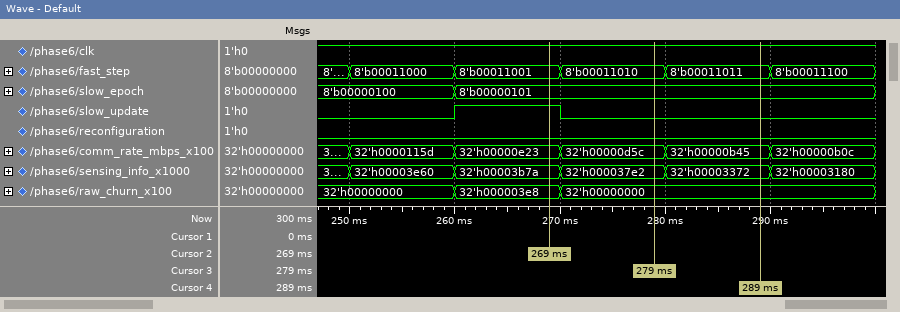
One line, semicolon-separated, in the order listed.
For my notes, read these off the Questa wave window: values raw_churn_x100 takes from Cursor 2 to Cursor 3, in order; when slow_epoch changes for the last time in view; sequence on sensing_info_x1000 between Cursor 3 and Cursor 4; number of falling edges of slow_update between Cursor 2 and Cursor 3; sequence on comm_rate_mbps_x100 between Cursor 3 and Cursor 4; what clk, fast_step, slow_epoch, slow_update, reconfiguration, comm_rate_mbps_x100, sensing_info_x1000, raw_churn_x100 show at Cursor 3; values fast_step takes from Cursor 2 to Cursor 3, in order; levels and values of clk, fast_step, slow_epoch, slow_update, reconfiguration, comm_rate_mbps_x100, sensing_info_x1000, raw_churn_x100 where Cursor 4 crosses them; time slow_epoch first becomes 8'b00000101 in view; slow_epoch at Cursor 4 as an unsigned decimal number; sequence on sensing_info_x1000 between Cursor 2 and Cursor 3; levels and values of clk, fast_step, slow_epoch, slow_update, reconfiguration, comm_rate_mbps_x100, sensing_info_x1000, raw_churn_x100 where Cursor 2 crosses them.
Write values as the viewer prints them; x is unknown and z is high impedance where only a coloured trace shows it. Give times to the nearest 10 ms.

32'h000003e8, 32'h00000000; 260 ms; 32'h000037e2, 32'h00003372; 1; 32'h00000d5c, 32'h00000b45; clk=1, fast_step=8'b00011010, slow_epoch=8'b00000101, slow_update=0, reconfiguration=0, comm_rate_mbps_x100=32'h00000d5c, sensing_info_x1000=32'h000037e2, raw_churn_x100=32'h00000000; 8'b00011001, 8'b00011010; clk=1, fast_step=8'b00011011, slow_epoch=8'b00000101, slow_update=0, reconfiguration=0, comm_rate_mbps_x100=32'h00000b45, sensing_info_x1000=32'h00003372, raw_churn_x100=32'h00000000; 260 ms; 5; 32'h00003b7a, 32'h000037e2; clk=1, fast_step=8'b00011001, slow_epoch=8'b00000101, slow_update=1, reconfiguration=0, comm_rate_mbps_x100=32'h00000e23, sensing_info_x1000=32'h00003b7a, raw_churn_x100=32'h000003e8
